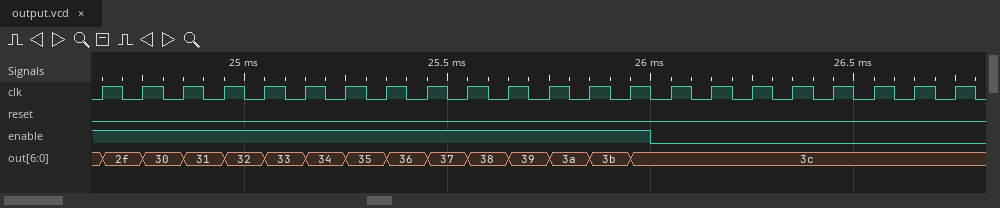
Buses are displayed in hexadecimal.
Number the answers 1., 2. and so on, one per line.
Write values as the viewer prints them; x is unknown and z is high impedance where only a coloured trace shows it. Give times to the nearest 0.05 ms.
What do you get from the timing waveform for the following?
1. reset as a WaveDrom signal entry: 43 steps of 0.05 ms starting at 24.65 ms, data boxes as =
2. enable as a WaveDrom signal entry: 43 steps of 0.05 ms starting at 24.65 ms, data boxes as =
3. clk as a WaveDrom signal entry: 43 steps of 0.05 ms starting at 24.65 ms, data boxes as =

1. {name: 'reset', wave: '0..........................................'}
2. {name: 'enable', wave: '1..........................0...............'}
3. {name: 'clk', wave: '1010101010101010101010101010101010101010101'}
